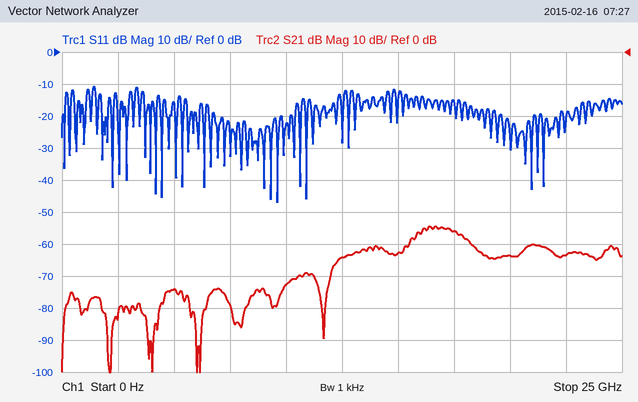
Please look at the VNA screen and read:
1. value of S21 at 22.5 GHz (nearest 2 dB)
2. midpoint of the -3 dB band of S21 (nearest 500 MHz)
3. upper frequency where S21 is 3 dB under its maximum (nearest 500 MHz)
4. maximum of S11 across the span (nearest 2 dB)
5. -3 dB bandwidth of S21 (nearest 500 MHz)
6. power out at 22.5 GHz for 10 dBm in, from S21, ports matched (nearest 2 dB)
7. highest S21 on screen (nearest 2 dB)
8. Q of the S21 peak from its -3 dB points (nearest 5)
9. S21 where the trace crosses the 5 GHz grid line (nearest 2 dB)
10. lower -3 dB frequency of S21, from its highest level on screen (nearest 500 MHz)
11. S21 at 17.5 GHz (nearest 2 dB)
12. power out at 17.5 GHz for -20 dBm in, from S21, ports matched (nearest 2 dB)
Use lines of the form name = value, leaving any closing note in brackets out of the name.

value of S21 at 22.5 GHz = -64 dB
midpoint of the -3 dB band of S21 = 17.0 GHz
upper frequency where S21 is 3 dB under its maximum = 18.0 GHz
maximum of S11 across the span = -10 dB
-3 dB bandwidth of S21 = 2.0 GHz
power out at 22.5 GHz for 10 dBm in, from S21, ports matched = -54 dBm
highest S21 on screen = -54 dB
Q of the S21 peak from its -3 dB points = 10
S21 where the trace crosses the 5 GHz grid line = -74 dB
lower -3 dB frequency of S21, from its highest level on screen = 16.0 GHz
S21 at 17.5 GHz = -56 dB
power out at 17.5 GHz for -20 dBm in, from S21, ports matched = -76 dBm
